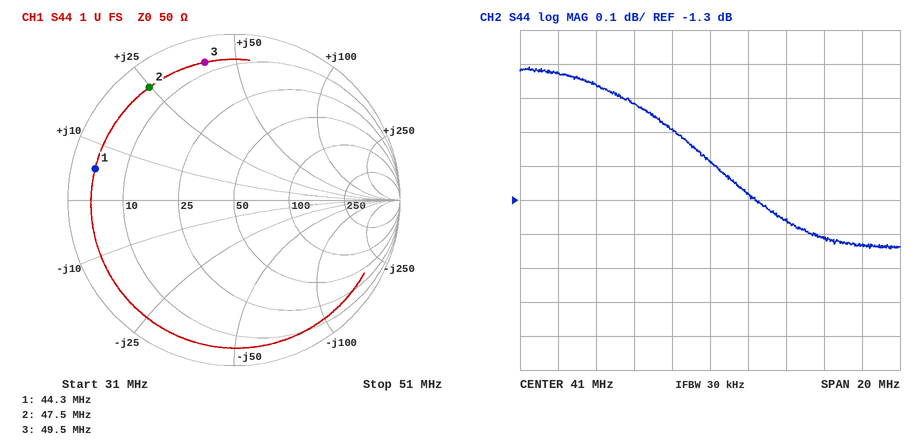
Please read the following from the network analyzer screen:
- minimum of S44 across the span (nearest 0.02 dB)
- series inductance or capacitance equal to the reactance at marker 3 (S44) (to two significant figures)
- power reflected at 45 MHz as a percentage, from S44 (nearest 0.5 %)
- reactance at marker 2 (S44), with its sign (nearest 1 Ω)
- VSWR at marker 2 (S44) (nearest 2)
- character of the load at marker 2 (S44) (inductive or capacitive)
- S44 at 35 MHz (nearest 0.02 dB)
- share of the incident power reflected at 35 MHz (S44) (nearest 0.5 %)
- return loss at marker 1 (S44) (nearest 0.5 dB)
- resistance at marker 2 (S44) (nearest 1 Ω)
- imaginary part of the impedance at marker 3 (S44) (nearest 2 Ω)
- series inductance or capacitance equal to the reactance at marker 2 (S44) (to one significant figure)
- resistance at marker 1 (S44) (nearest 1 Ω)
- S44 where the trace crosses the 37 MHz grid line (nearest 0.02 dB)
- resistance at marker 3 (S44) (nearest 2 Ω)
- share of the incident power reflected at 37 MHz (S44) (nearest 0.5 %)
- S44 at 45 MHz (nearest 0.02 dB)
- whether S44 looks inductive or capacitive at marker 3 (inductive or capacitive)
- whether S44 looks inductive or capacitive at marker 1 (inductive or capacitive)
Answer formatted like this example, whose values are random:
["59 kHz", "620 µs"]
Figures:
["-1.44 dB", "130 nH", "73.0 %", "+25 Ω", "12", "inductive", "-0.96 dB", "80.0 %", "1.5 dB", "5 Ω", "+40 Ω", "80 nH", "4 Ω", "-1.02 dB", "6 Ω", "79.0 %", "-1.36 dB", "inductive", "inductive"]
